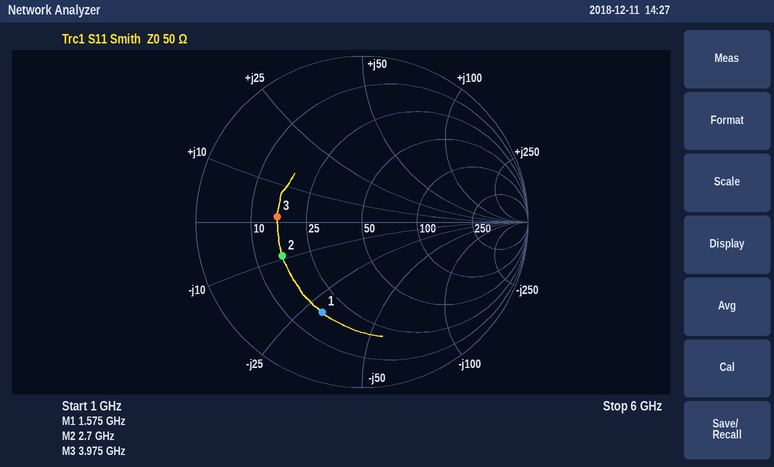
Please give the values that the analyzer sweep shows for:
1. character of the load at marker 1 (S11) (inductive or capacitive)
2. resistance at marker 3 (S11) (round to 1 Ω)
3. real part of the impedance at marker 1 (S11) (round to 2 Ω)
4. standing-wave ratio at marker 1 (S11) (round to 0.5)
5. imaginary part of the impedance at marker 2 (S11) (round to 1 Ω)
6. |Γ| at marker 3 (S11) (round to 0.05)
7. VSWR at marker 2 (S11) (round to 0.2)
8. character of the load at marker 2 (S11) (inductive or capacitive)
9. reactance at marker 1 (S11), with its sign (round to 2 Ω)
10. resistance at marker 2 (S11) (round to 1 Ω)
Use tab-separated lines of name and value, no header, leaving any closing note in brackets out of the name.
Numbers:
character of the load at marker 1 (S11)	capacitive
resistance at marker 3 (S11)	16 Ω
real part of the impedance at marker 1 (S11)	18 Ω
standing-wave ratio at marker 1 (S11)	4.0
imaginary part of the impedance at marker 2 (S11)	-9 Ω
|Γ| at marker 3 (S11)	0.50
VSWR at marker 2 (S11)	3.2
character of the load at marker 2 (S11)	capacitive
reactance at marker 1 (S11), with its sign	-30 Ω
resistance at marker 2 (S11)	16 Ω
